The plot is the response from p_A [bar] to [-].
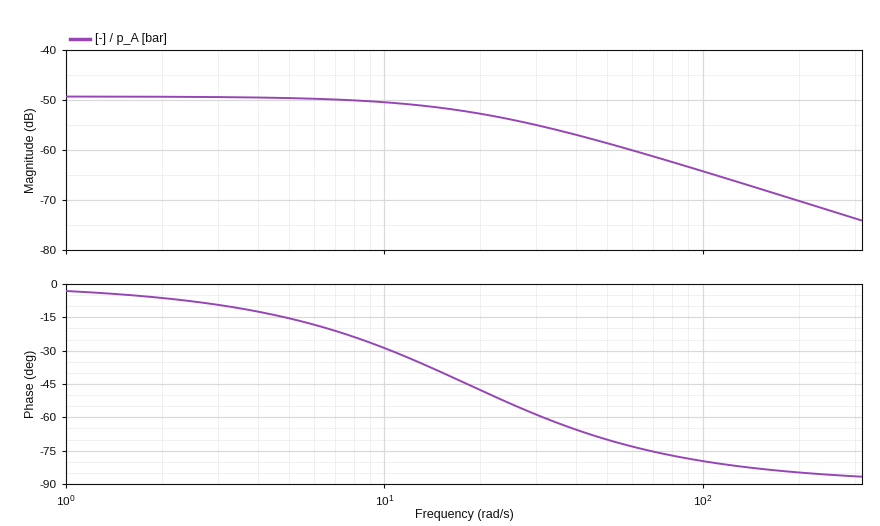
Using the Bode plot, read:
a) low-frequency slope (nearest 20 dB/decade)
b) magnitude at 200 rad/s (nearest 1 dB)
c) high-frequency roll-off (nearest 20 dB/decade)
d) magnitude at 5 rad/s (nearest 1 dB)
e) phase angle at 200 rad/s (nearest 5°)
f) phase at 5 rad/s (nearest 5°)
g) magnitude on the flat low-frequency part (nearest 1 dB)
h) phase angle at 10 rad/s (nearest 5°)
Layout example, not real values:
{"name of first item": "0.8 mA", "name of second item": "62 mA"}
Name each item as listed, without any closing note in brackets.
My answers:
{"low-frequency slope": "0 dB/decade", "magnitude at 200 rad/s": "-70 dB", "high-frequency roll-off": "-20 dB/decade", "magnitude at 5 rad/s": "-50 dB", "phase angle at 200 rad/s": "-85°", "phase at 5 rad/s": "-15°", "magnitude on the flat low-frequency part": "-49 dB", "phase angle at 10 rad/s": "-30°"}
